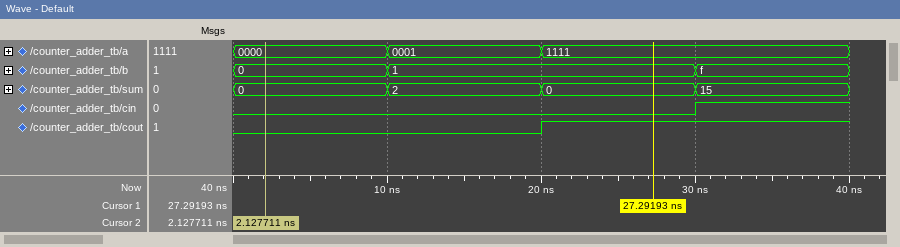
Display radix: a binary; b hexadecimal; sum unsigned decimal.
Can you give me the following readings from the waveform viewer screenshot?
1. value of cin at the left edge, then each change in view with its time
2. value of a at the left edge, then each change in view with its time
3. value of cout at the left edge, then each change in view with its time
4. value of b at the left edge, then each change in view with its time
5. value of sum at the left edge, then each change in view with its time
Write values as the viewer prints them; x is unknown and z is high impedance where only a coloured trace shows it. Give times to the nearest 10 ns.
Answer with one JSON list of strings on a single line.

["0, 1 at 30 ns", "0000, 0001 at 10 ns, 1111 at 20 ns", "0, 1 at 20 ns", "0, 1 at 10 ns, f at 30 ns", "0, 2 at 10 ns, 0 at 20 ns, 15 at 30 ns"]
